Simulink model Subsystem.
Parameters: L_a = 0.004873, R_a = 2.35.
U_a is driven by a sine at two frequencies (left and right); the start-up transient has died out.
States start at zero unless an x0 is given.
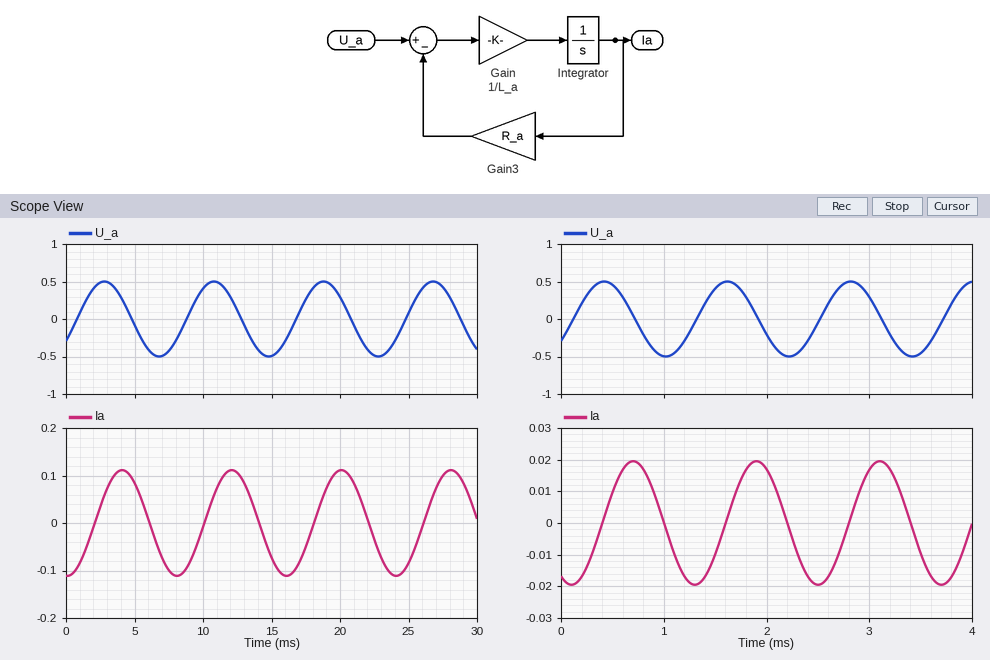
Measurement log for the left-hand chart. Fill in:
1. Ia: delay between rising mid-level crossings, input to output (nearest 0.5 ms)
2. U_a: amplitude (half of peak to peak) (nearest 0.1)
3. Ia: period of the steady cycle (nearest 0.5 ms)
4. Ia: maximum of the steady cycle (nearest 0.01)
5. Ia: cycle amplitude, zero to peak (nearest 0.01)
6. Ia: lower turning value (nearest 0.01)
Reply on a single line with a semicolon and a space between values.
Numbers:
1.5 ms; 0.5; 8.0 ms; 0.11; 0.11; -0.11
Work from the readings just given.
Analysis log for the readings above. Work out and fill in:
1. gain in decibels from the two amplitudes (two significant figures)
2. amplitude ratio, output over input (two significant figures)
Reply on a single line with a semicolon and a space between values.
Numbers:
-13 dB; 0.22
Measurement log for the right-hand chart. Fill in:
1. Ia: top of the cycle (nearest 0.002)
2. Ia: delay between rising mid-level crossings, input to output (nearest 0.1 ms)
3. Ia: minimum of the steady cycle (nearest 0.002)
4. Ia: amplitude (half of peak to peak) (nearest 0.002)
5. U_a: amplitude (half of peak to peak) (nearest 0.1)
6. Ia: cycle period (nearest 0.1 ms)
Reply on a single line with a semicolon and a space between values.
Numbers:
0.020; 0.3 ms; -0.020; 0.020; 0.5; 1.2 ms
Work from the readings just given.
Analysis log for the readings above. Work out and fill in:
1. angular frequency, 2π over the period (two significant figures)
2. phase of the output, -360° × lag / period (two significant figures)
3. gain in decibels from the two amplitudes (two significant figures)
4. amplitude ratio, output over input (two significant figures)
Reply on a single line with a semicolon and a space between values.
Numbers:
5.2 rad/ms; -90°; -28 dB; 0.040
